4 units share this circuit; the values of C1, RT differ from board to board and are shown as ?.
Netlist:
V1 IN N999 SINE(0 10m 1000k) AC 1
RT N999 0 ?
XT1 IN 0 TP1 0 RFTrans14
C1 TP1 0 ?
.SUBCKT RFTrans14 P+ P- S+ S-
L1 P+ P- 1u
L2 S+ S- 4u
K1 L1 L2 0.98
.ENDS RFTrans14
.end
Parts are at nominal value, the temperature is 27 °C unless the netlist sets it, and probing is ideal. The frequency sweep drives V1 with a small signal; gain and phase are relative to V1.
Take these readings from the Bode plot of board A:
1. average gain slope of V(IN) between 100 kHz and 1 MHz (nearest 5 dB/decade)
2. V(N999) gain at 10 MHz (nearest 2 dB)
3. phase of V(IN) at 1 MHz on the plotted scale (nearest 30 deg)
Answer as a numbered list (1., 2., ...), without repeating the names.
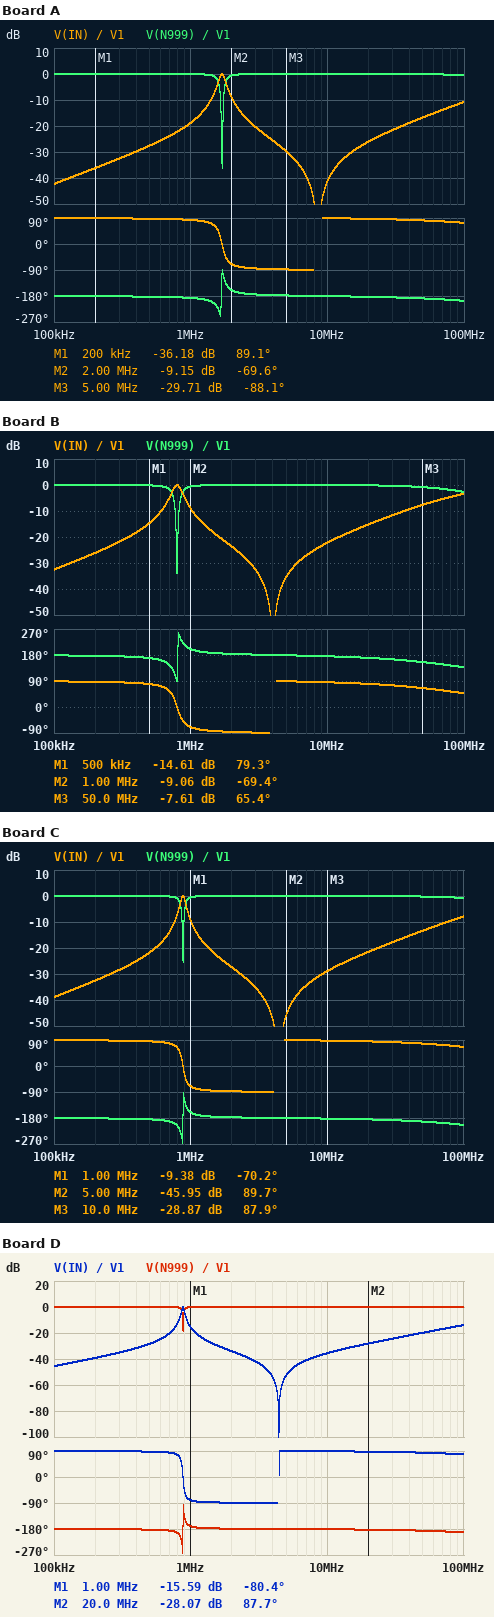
1. 25 dB/decade
2. 0 dB
3. 90 deg
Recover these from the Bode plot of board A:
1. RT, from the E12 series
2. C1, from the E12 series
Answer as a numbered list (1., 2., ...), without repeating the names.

1. 82 Ω
2. 2.2 nF
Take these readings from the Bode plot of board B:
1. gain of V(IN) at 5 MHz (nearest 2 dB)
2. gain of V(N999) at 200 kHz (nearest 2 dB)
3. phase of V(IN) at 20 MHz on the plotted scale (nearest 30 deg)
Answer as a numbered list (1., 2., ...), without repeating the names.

1. -36 dB
2. 0 dB
3. 90 deg
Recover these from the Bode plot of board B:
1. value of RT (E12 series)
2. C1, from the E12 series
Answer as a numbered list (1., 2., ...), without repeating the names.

1. 27 Ω
2. 10 nF
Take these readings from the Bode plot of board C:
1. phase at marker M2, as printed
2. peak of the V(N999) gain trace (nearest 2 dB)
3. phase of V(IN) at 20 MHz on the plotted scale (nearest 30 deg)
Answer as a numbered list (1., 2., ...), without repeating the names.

1. 89.7 deg
2. 0 dB
3. 90 deg
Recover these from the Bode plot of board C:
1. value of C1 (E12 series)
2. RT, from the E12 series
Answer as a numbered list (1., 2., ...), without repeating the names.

1. 8.2 nF
2. 56 Ω
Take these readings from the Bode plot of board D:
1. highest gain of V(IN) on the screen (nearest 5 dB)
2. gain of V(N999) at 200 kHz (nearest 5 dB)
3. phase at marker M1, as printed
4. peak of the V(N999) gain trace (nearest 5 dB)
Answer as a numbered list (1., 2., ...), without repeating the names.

1. 0 dB
2. 0 dB
3. -80.4 deg
4. 0 dB
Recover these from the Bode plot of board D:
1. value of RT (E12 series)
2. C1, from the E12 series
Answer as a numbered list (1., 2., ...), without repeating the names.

1. 120 Ω
2. 8.2 nF
